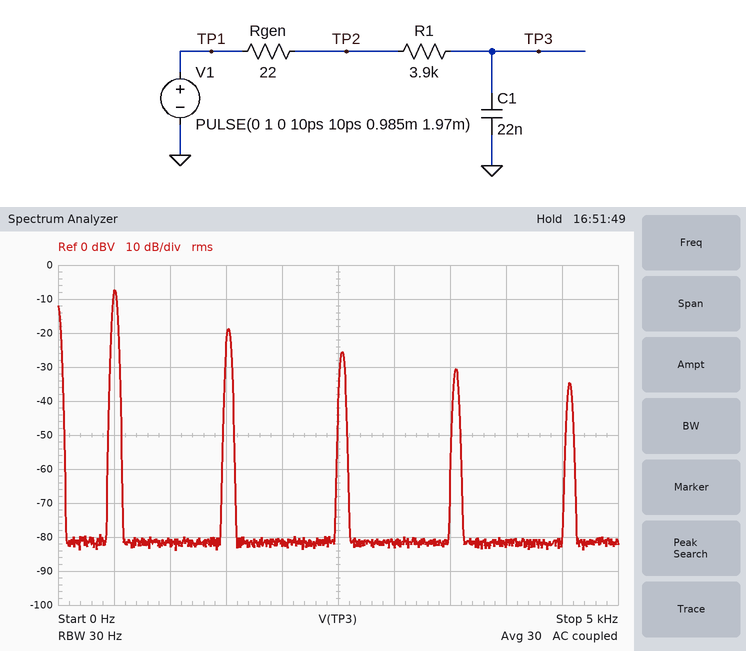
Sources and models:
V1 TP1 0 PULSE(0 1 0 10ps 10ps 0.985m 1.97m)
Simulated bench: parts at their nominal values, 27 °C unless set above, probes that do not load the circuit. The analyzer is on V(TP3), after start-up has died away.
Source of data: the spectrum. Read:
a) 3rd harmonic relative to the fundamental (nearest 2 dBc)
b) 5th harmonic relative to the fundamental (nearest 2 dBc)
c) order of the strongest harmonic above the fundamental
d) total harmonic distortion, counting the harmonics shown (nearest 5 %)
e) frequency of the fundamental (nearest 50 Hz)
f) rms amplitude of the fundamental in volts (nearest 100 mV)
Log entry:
-12 dBc
-18 dBc
3
30 %
500 Hz
400 mV
